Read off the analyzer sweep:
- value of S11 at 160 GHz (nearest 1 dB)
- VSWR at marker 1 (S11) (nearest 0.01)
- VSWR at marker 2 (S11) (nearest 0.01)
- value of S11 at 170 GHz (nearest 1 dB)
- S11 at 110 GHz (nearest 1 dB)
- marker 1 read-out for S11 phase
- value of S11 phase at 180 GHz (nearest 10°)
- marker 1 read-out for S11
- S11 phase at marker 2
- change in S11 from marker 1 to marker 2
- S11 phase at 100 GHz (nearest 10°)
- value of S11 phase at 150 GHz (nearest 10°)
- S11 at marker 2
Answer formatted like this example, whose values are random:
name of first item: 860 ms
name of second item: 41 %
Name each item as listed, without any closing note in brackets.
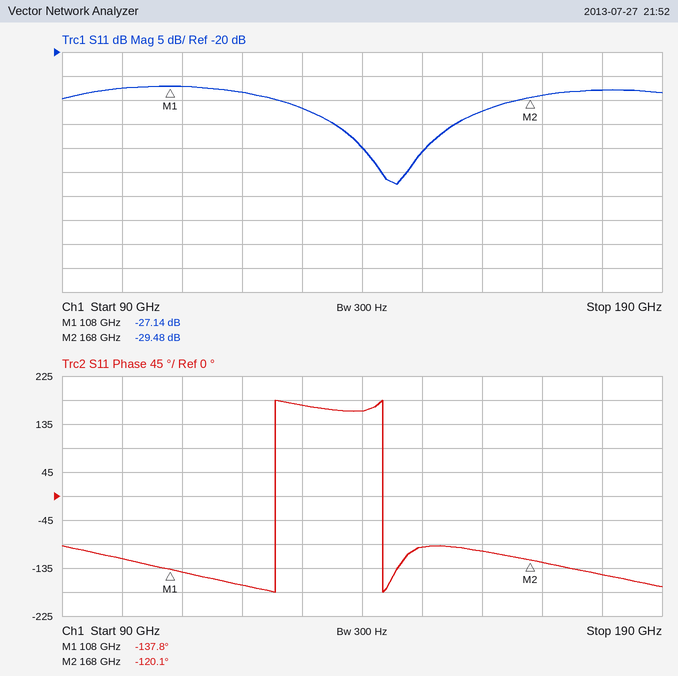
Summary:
value of S11 at 160 GHz: -32 dB
VSWR at marker 1 (S11): 1.09
VSWR at marker 2 (S11): 1.07
value of S11 at 170 GHz: -29 dB
S11 at 110 GHz: -27 dB
marker 1 read-out for S11 phase: -137.8°
value of S11 phase at 180 GHz: -150°
marker 1 read-out for S11: -27.14 dB
S11 phase at marker 2: -120.1°
change in S11 from marker 1 to marker 2: -2.34 dB
S11 phase at 100 GHz: -120°
value of S11 phase at 150 GHz: -100°
S11 at marker 2: -29.48 dB
